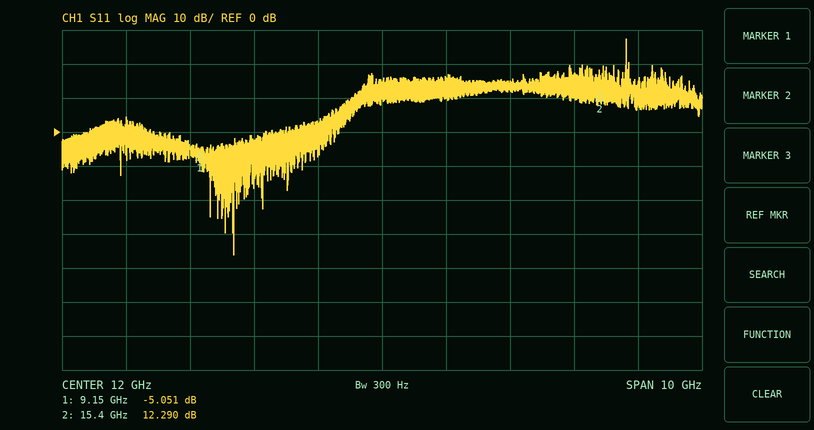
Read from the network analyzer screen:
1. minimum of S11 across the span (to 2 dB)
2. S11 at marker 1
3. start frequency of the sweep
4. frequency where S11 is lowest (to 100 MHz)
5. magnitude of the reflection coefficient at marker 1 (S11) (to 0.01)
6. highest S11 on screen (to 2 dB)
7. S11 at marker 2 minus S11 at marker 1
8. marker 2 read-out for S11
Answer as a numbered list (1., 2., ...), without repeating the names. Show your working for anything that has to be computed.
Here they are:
1. -36 dB
2. -5.051 dB
3. 7 GHz
4. 9.7 GHz
5. 10^(-5.051/20) ≈ 0.56
6. 28 dB
7. 12.29 − (-5.051) = 17.341 dB
8. 12.290 dB
